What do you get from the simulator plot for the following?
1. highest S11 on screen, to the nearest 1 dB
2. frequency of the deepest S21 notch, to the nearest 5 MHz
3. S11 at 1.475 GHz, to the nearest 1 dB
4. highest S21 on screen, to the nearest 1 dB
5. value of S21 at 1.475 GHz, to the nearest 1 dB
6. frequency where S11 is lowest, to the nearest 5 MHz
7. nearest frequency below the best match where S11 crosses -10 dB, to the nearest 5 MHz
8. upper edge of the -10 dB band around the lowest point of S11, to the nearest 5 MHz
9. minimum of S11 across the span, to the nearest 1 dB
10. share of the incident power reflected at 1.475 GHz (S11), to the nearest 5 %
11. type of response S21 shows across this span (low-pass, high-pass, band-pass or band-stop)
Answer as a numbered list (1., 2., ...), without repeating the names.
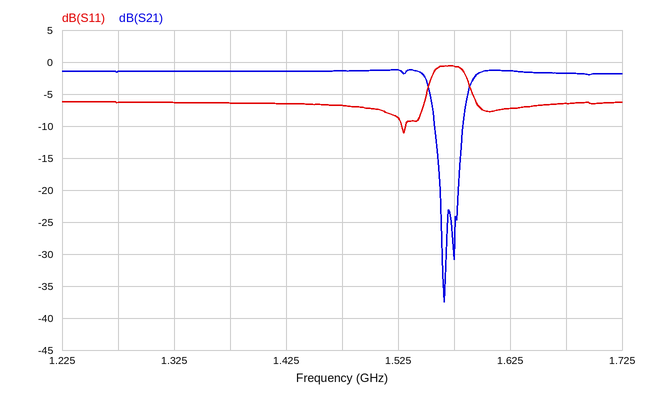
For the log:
1. -1 dB
2. 1.565 GHz
3. -7 dB
4. -1 dB
5. -1 dB
6. 1.530 GHz
7. 1.530 GHz
8. 1.530 GHz
9. -11 dB
10. 20 %
11. band-stop
